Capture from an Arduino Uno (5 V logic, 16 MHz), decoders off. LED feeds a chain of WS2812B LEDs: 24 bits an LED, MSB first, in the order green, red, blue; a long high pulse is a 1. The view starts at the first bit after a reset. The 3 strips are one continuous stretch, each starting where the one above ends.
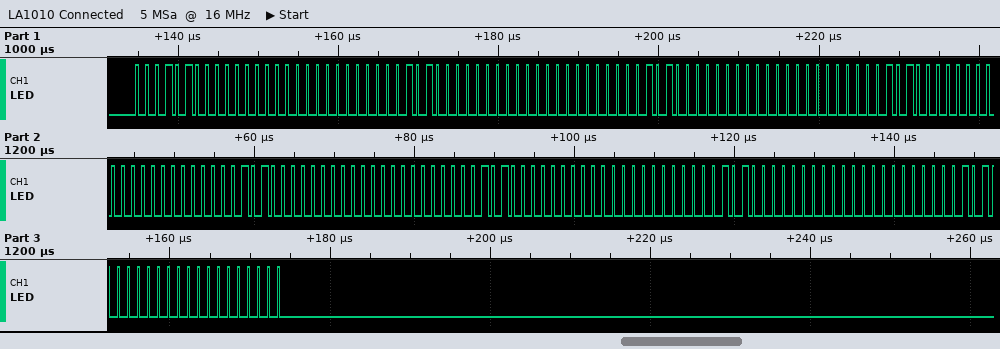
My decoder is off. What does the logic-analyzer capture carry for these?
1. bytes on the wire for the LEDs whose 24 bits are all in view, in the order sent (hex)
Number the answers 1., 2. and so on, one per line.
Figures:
1. 14 00 00 14 00 00 14 00 00 14 00 00 14 00 00 14 00 00 14 00 00 14 00 00
